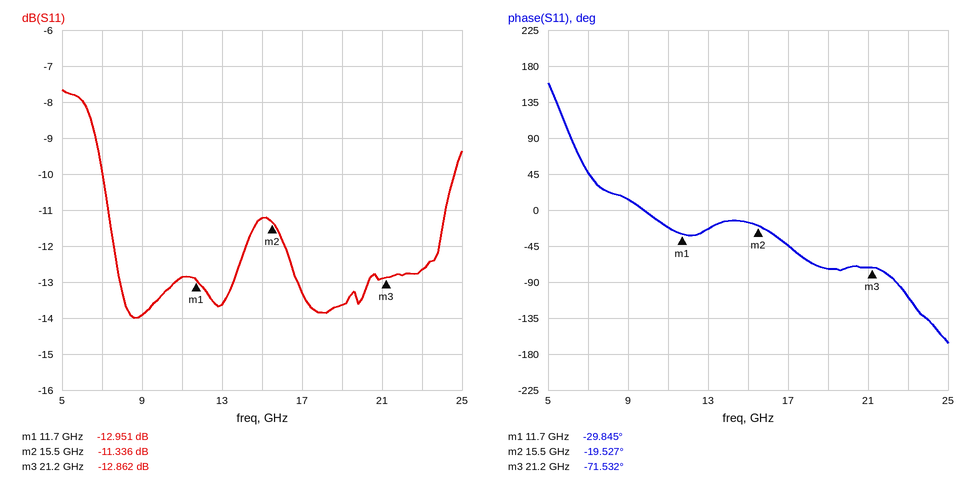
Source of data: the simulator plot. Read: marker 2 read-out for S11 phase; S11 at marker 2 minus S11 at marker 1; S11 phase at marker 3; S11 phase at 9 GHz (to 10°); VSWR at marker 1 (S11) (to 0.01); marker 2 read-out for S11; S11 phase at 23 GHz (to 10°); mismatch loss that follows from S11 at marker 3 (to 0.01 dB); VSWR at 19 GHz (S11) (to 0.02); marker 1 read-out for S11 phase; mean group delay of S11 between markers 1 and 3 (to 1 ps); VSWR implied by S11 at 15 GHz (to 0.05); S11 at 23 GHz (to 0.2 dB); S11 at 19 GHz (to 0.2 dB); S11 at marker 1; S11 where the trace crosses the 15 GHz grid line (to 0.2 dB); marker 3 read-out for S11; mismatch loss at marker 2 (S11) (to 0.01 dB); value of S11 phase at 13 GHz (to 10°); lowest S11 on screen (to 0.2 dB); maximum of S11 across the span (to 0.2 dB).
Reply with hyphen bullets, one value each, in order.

- -19.527°
- 1.615 dB
- -71.532°
- 10°
- 1.58
- -11.336 dB
- -110°
- 0.23 dB
- 1.52
- -29.845°
- 12 ps
- 1.75
- -12.6 dB
- -13.6 dB
- -12.951 dB
- -11.2 dB
- -12.862 dB
- 0.33 dB
- -20°
- -14.0 dB
- -7.6 dB
